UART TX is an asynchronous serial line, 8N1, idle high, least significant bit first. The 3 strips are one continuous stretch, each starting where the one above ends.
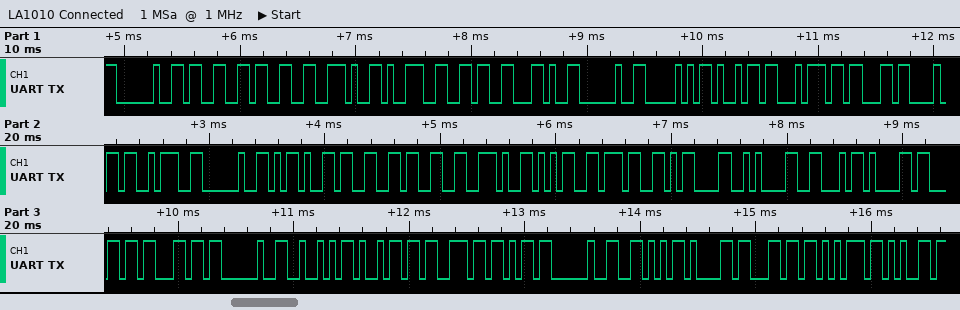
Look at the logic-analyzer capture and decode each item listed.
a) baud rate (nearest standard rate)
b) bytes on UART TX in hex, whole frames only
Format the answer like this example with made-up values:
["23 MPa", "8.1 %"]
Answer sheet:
["19200 baud", "20 33 33 2E 39 36 2C 20 50 69 74 63 68 3A 20 2D 33 33 2E 35 37 0D 0A 46 61 6C 6C 20 52 69 73 6B 20 56 61 6C 75 65"]
